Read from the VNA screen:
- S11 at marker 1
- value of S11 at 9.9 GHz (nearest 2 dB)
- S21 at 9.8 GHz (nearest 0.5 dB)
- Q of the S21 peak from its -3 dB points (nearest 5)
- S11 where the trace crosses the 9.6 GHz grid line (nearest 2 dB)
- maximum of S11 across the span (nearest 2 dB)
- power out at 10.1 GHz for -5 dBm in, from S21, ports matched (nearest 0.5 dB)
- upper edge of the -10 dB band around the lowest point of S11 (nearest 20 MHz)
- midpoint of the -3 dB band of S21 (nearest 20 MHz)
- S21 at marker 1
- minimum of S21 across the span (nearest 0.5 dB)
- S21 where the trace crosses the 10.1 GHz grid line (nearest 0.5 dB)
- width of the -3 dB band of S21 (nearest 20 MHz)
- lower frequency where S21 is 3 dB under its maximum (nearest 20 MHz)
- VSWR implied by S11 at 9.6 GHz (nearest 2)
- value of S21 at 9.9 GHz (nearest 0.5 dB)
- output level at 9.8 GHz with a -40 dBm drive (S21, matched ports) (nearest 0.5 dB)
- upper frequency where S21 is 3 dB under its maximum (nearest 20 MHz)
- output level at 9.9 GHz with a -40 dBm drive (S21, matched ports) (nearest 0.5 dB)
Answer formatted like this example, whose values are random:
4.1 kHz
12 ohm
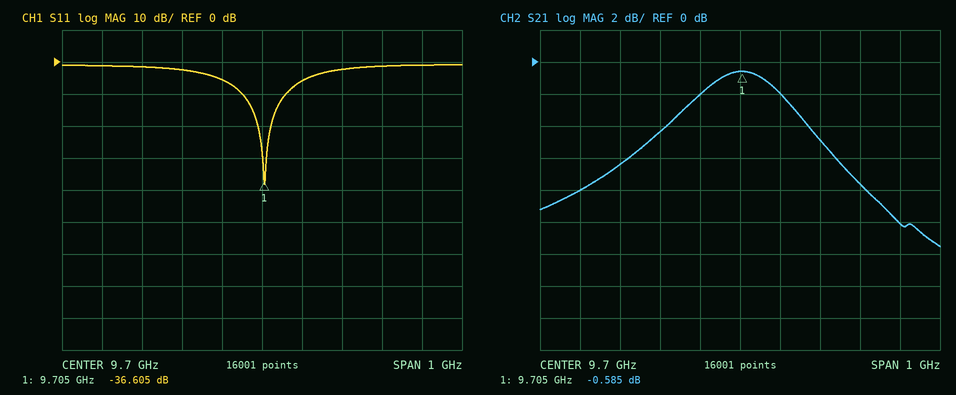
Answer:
-36.605 dB
-2 dB
-2.0 dB
30
-6 dB
0 dB
-15.0 dBm
9.76 GHz
9.70 GHz
-0.585 dB
-11.5 dB
-10.0 dB
320 MHz
9.54 GHz
4
-5.0 dB
-42.0 dBm
9.86 GHz
-45.0 dBm
